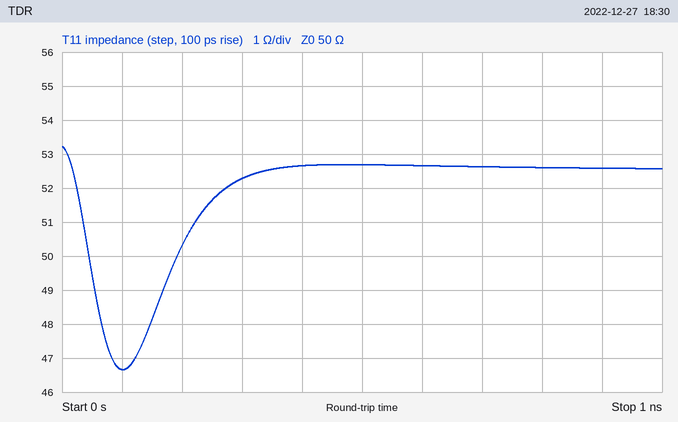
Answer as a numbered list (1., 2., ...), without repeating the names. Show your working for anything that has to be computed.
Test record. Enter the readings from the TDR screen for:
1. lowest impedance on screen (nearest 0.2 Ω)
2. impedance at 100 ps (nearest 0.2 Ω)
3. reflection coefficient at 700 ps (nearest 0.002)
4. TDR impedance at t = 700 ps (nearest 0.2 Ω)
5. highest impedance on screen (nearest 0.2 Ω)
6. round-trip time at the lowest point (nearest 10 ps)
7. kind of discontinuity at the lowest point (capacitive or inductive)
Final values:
1. 46.6 Ω
2. 46.6 Ω
3. (52.6 − 50)/(52.6 + 50) ≈ +0.0253, so +0.026 to the nearest 0.002
4. 52.6 Ω
5. 53.2 Ω
6. 100 ps
7. capacitive
